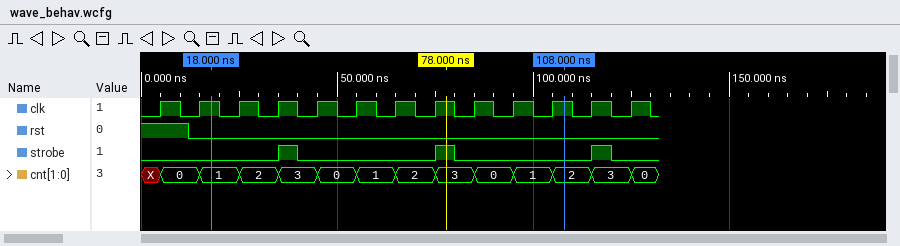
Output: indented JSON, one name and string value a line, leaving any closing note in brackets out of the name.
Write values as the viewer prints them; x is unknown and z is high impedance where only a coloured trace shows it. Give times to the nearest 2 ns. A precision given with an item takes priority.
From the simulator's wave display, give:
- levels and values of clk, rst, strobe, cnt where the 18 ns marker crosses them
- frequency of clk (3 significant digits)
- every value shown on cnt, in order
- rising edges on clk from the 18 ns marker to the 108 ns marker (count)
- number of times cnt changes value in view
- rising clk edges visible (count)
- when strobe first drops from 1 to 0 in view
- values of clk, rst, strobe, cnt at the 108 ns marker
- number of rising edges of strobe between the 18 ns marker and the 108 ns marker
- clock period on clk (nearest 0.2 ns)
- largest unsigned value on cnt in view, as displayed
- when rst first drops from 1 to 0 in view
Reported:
{
  "levels and values of clk, rst, strobe, cnt where the 18 ns marker crosses them": "clk=1, rst=0, strobe=0, cnt=1",
  "frequency of clk": "100 MHz",
  "every value shown on cnt, in order": "X, 0, 1, 2, 3, 0, 1, 2, 3, 0, 1, 2, 3, 0",
  "rising edges on clk from the 18 ns marker to the 108 ns marker": "9",
  "number of times cnt changes value in view": "13",
  "rising clk edges visible": "13",
  "when strobe first drops from 1 to 0 in view": "40 ns",
  "values of clk, rst, strobe, cnt at the 108 ns marker": "clk=1, rst=0, strobe=0, cnt=2",
  "number of rising edges of strobe between the 18 ns marker and the 108 ns marker": "2",
  "clock period on clk": "10 ns",
  "largest unsigned value on cnt in view, as displayed": "3",
  "when rst first drops from 1 to 0 in view": "12 ns"
}
